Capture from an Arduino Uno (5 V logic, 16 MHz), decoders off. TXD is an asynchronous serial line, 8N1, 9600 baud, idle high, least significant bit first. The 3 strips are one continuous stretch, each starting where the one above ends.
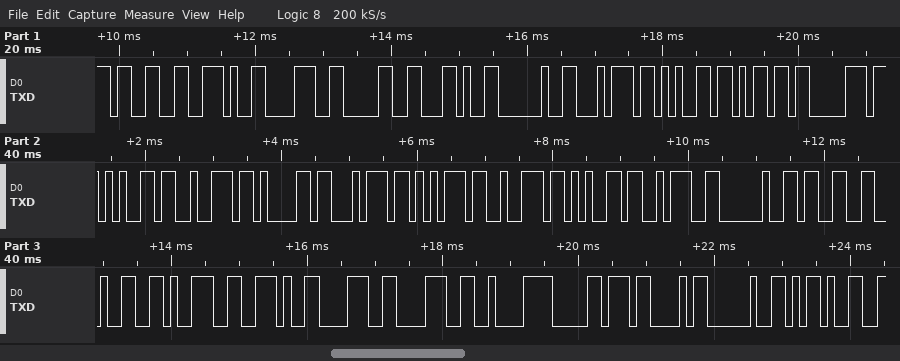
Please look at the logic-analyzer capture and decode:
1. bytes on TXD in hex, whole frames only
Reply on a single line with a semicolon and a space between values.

33 2E 38 30 2C 20 74 65 6D 70 65 72 61 74 75 72 65 3A 20 33 32 39 2E 38 38 C2 B0 43 20 2D
